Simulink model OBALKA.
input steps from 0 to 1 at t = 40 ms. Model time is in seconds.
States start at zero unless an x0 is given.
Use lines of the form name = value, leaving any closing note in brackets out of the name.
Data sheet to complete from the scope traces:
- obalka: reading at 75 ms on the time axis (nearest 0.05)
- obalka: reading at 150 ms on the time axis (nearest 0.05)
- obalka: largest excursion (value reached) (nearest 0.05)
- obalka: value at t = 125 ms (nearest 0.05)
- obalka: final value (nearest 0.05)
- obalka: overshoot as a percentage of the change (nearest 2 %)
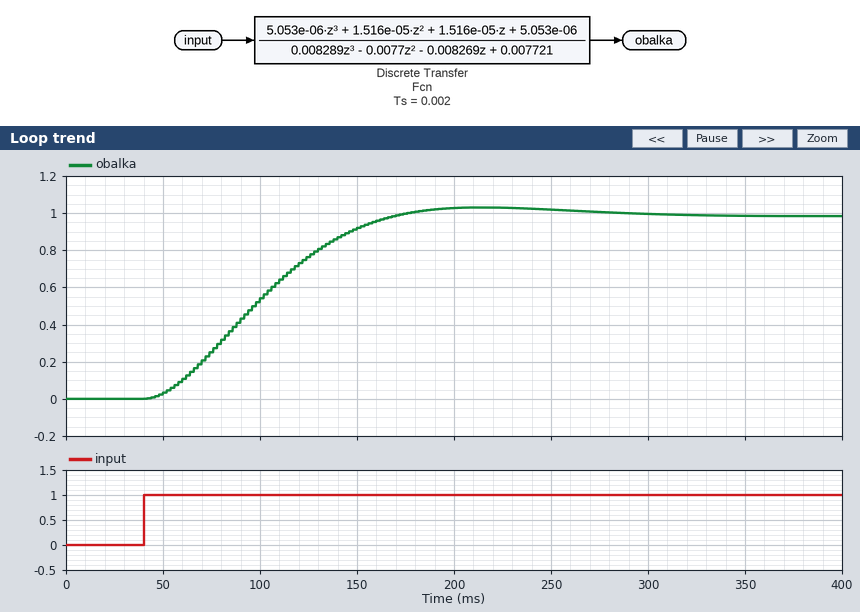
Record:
obalka: reading at 75 ms on the time axis = 0.25
obalka: reading at 150 ms on the time axis = 0.90
obalka: largest excursion (value reached) = 1.05
obalka: value at t = 125 ms = 0.75
obalka: final value = 1.00
obalka: overshoot as a percentage of the change = 4 %
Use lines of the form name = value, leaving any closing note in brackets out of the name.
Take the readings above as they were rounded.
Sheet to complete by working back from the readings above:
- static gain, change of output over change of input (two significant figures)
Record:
static gain, change of output over change of input = 1.0
